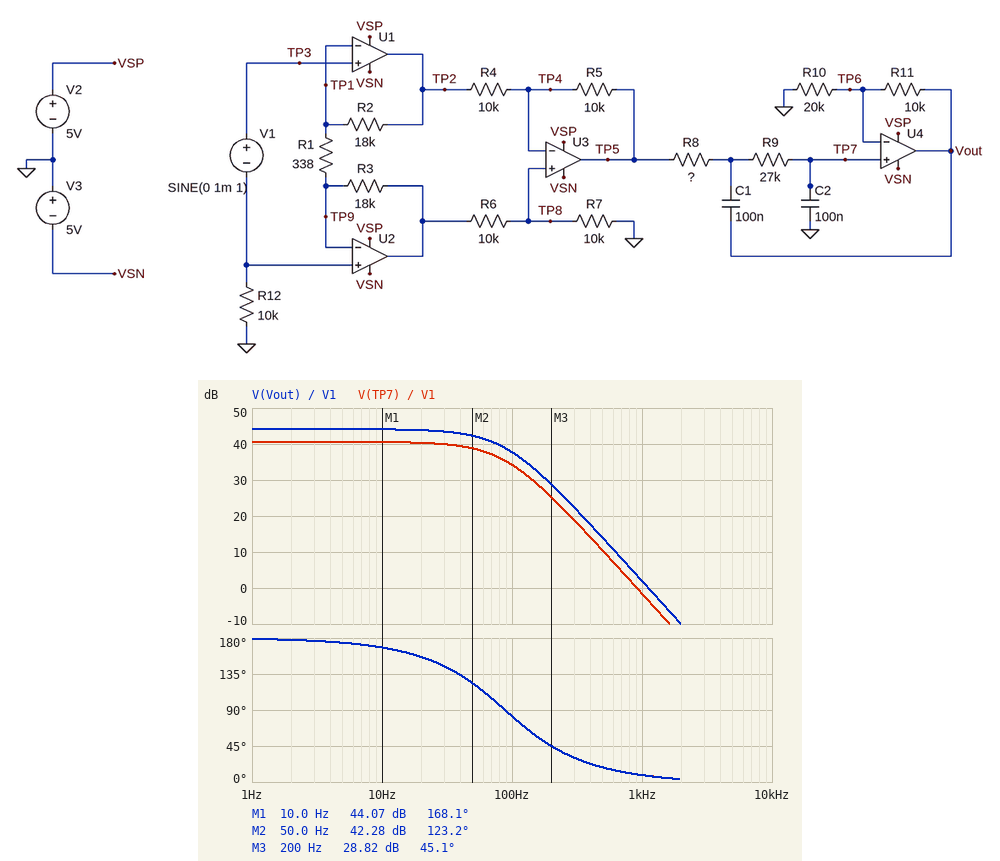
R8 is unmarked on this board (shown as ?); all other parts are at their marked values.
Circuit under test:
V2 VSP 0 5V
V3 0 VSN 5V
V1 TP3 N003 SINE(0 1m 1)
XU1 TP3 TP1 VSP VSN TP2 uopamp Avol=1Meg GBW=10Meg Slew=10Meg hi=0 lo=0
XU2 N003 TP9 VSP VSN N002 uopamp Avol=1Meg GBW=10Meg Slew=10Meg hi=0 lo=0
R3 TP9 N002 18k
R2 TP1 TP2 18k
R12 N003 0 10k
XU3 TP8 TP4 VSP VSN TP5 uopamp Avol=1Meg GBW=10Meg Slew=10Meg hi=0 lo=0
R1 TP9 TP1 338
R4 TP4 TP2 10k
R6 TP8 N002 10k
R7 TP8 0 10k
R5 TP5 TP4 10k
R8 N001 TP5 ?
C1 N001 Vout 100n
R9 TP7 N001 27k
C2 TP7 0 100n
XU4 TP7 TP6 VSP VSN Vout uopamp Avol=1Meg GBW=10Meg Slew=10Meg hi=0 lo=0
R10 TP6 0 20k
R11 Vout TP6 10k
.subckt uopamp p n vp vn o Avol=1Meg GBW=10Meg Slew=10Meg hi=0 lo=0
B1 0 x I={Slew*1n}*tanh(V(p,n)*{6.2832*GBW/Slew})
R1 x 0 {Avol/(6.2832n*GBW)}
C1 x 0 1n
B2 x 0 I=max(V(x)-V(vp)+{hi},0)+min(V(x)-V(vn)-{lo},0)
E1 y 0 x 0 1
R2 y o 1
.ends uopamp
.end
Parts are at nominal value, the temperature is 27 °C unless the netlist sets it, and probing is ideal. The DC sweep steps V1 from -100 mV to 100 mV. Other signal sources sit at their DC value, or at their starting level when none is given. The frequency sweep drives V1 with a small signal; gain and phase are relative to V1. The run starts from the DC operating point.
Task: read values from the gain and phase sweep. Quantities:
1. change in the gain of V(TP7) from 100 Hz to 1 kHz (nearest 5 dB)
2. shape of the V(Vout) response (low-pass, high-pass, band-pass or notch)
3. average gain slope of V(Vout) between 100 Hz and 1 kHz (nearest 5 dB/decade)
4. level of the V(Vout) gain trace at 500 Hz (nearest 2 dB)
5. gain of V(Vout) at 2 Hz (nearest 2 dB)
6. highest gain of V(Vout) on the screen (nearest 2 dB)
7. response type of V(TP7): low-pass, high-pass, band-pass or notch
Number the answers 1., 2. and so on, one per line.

1. -35 dB
2. low-pass
3. -35 dB/decade
4. 14 dB
5. 44 dB
6. 44 dB
7. low-pass
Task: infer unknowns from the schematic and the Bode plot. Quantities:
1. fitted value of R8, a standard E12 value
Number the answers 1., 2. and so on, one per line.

1. 12 kΩ
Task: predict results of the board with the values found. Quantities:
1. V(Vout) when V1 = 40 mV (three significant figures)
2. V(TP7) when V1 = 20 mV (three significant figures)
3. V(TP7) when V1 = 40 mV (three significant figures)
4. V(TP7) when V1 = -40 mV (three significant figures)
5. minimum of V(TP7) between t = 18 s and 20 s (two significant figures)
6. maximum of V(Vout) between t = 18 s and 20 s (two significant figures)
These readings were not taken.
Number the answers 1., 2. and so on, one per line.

1. -5.01 V
2. -2.15 V
3. -4.30 V
4. 4.30 V
5. -110 mV
6. 160 mV
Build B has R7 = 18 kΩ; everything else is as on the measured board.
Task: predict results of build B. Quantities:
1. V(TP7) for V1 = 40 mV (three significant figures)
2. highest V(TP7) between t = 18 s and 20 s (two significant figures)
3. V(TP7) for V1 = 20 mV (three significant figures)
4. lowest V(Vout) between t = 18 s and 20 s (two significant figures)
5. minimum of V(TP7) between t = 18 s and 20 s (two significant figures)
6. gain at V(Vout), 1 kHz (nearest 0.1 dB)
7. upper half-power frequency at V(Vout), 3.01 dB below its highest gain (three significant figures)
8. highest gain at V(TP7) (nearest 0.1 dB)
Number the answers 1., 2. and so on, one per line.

1. -4.91 V
2. 120 mV
3. -2.45 V
4. -180 mV
5. -120 mV
6. 3.1 dB
7. 64.3 Hz
8. 41.8 dB
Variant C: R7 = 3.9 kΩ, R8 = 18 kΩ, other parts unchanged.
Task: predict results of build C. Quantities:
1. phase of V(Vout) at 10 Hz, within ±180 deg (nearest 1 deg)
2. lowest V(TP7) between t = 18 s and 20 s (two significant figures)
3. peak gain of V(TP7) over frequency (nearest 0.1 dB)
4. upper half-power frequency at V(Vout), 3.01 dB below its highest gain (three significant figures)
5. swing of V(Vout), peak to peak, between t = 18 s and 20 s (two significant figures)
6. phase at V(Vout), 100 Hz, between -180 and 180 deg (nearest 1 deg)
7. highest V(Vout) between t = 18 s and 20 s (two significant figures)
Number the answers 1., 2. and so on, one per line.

1. 167 deg
2. -84 mV
3. 38.5 dB
4. 61.3 Hz
5. 250 mV
6. 68 deg
7. 130 mV
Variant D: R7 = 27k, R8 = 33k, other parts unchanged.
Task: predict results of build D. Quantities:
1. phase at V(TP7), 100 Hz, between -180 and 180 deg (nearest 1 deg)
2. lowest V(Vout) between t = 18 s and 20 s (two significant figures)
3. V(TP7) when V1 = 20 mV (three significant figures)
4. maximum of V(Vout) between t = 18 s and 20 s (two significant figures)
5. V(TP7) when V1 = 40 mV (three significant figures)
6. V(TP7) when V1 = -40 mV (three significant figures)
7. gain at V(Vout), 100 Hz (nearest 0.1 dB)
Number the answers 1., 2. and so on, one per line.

1. 47 deg
2. -200 mV
3. -2.64 V
4. 200 mV
5. -5.01 V
6. 5.01 V
7. 34.5 dB
